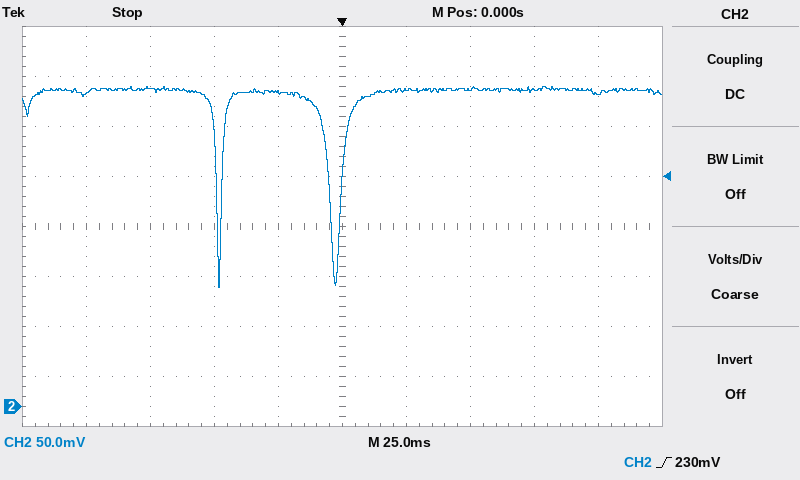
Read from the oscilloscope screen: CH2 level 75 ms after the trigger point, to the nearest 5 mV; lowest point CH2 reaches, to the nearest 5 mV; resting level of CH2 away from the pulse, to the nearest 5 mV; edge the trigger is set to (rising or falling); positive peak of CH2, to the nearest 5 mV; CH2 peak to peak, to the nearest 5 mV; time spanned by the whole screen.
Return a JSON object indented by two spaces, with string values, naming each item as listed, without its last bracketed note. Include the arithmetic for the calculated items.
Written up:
{
  "CH2 level 75 ms after the trigger point, to the nearest 5 mV": "315 mV",
  "lowest point CH2 reaches, to the nearest 5 mV": "120 mV",
  "resting level of CH2 away from the pulse, to the nearest 5 mV": "315 mV",
  "edge the trigger is set to": "rising",
  "positive peak of CH2, to the nearest 5 mV": "320 mV",
  "CH2 peak to peak, to the nearest 5 mV": "320 mV − (120 mV) = 200 mV",
  "time spanned by the whole screen": "250 ms"
}
